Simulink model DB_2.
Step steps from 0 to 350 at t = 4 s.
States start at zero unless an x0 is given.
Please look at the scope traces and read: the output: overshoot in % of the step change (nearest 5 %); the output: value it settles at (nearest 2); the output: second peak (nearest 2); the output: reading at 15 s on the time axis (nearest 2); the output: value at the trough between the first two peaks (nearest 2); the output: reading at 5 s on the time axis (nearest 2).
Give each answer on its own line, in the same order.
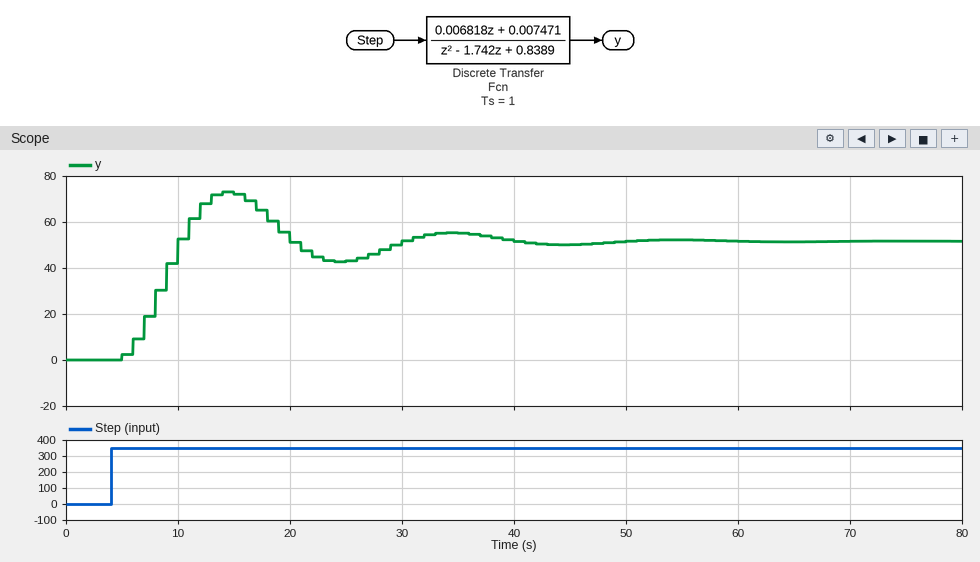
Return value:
40 %
52
56
72
42
2
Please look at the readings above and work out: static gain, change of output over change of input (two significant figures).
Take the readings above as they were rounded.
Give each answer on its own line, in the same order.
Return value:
0.15
